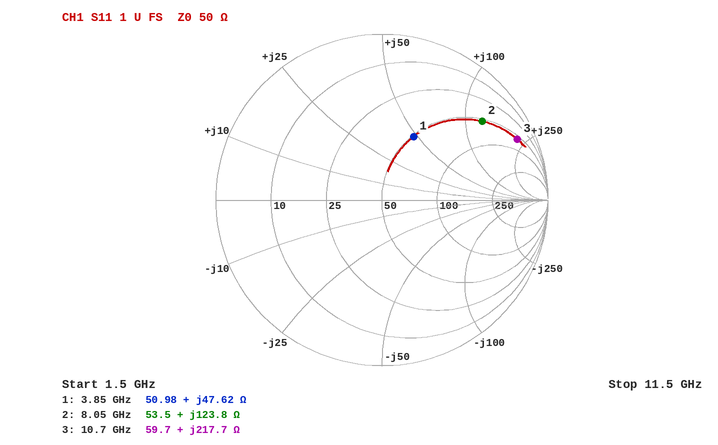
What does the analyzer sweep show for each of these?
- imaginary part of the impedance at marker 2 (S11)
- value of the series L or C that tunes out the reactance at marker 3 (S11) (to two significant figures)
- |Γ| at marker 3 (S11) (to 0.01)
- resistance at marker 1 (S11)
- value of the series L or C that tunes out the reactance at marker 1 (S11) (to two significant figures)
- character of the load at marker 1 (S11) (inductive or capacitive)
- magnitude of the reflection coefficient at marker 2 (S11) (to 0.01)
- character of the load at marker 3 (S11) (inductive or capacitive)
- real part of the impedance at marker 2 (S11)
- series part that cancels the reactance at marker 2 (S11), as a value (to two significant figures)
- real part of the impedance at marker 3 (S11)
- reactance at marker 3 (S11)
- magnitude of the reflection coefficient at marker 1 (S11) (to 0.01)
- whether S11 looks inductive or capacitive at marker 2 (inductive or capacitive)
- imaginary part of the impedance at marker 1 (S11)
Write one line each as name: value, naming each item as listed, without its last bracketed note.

imaginary part of the impedance at marker 2: +123.8 Ω
value of the series L or C that tunes out the reactance at marker 3 (S11): 68 fF
|Γ| at marker 3 (S11): 0.89
resistance at marker 1: 50.98 Ω
value of the series L or C that tunes out the reactance at marker 1 (S11): 870 fF
character of the load at marker 1 (S11): inductive
magnitude of the reflection coefficient at marker 2 (S11): 0.77
character of the load at marker 3 (S11): inductive
real part of the impedance at marker 2: 53.5 Ω
series part that cancels the reactance at marker 2 (S11), as a value: 160 fF
real part of the impedance at marker 3: 59.7 Ω
reactance at marker 3: +217.7 Ω
magnitude of the reflection coefficient at marker 1 (S11): 0.43
whether S11 looks inductive or capacitive at marker 2: inductive
imaginary part of the impedance at marker 1: +47.62 Ω
